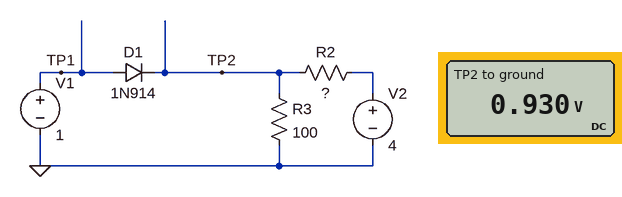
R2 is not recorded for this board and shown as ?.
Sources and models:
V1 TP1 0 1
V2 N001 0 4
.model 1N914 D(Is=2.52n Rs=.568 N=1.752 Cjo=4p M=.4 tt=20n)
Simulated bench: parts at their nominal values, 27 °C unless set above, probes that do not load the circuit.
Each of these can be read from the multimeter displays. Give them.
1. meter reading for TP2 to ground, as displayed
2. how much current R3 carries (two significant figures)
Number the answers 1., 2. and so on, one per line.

1. 0.930 V
2. 9.3 mA
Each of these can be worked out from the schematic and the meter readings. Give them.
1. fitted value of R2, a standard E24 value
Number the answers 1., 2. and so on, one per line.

1. 330 Ω
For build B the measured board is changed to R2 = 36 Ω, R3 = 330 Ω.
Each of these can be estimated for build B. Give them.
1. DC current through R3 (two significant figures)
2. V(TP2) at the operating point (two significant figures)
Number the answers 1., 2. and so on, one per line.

1. 11 mA
2. 3.6 V
